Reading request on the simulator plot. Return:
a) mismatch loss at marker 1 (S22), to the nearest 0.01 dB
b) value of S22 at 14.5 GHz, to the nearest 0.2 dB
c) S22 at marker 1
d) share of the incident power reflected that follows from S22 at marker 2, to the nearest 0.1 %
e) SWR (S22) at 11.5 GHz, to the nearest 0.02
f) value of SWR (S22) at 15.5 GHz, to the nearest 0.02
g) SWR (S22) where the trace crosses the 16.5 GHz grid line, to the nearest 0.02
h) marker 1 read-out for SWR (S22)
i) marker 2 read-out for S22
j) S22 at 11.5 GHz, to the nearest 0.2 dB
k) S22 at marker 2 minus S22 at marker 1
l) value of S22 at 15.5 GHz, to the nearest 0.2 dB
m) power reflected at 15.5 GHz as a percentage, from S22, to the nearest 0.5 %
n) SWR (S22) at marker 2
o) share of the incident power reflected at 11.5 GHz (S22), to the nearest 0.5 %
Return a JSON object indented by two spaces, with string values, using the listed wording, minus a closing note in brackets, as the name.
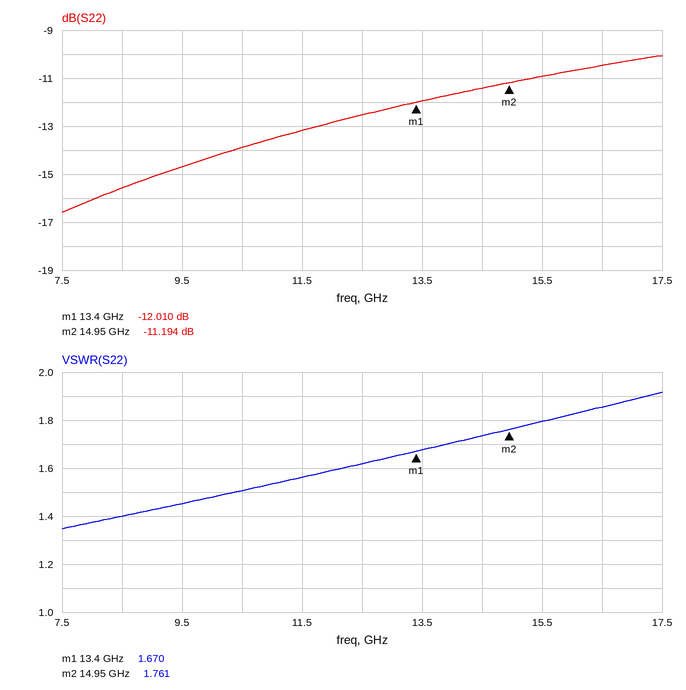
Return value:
{
  "mismatch loss at marker 1 (S22), to the nearest 0.01 dB": "0.28 dB",
  "value of S22 at 14.5 GHz, to the nearest 0.2 dB": "-11.4 dB",
  "S22 at marker 1": "-12.010 dB",
  "share of the incident power reflected that follows from S22 at marker 2, to the nearest 0.1 %": "7.6 %",
  "SWR (S22) at 11.5 GHz, to the nearest 0.02": "1.56",
  "value of SWR (S22) at 15.5 GHz, to the nearest 0.02": "1.80",
  "SWR (S22) where the trace crosses the 16.5 GHz grid line, to the nearest 0.02": "1.86",
  "marker 1 read-out for SWR": "1.670",
  "marker 2 read-out for S22": "-11.194 dB",
  "S22 at 11.5 GHz, to the nearest 0.2 dB": "-13.2 dB",
  "S22 at marker 2 minus S22 at marker 1": "0.816 dB",
  "value of S22 at 15.5 GHz, to the nearest 0.2 dB": "-11.0 dB",
  "power reflected at 15.5 GHz as a percentage, from S22, to the nearest 0.5 %": "8.0 %",
  "SWR (S22) at marker 2": "1.761",
  "share of the incident power reflected at 11.5 GHz (S22), to the nearest 0.5 %": "5.0 %"
}
